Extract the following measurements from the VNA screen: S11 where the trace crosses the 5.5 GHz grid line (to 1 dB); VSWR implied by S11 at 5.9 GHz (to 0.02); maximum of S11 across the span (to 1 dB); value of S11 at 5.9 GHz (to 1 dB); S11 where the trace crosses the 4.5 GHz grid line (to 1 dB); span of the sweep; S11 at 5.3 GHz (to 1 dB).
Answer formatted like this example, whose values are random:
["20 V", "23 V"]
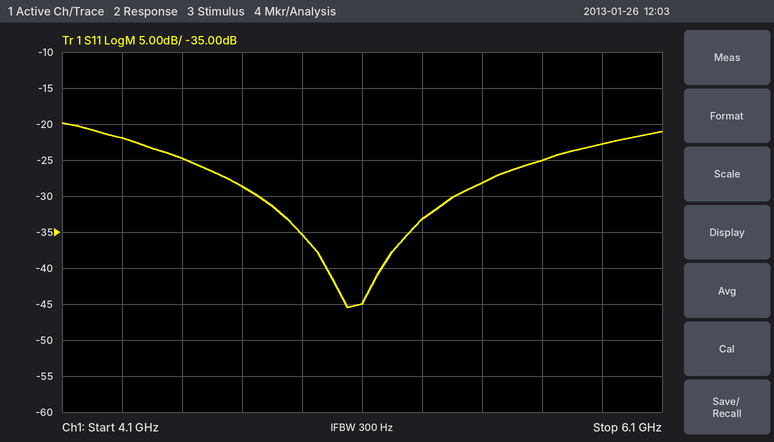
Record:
["-28 dB", "1.16", "-20 dB", "-23 dB", "-25 dB", "2 GHz", "-33 dB"]
